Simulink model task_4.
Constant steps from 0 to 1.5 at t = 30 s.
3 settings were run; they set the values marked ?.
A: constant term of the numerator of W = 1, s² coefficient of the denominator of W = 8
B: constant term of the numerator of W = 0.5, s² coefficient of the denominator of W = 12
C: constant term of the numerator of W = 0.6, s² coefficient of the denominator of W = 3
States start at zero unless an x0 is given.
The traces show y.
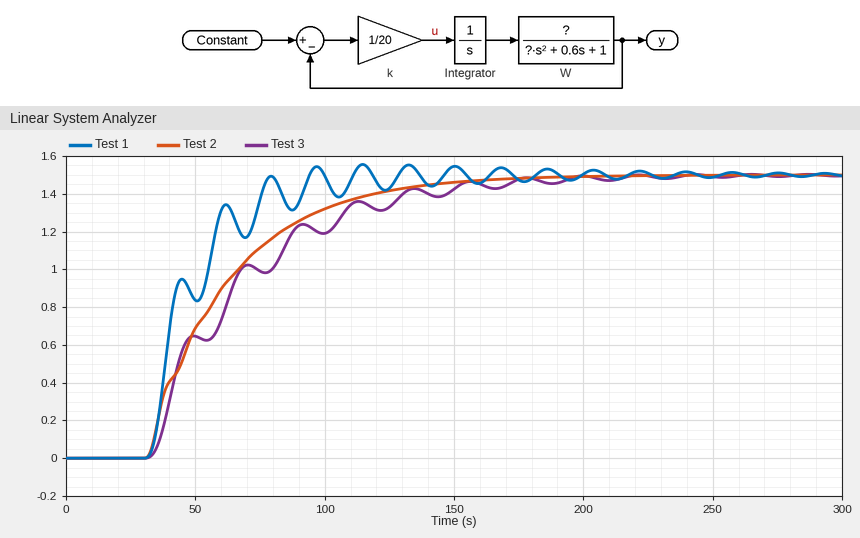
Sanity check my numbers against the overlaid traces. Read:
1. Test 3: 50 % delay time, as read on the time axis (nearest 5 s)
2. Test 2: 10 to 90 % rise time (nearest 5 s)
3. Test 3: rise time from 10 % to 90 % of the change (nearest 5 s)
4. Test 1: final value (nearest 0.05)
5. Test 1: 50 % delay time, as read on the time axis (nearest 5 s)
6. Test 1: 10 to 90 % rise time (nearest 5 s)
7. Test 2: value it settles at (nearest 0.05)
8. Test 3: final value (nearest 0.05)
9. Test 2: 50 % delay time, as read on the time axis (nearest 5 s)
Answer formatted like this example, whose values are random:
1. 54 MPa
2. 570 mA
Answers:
1. 60 s
2. 70 s
3. 75 s
4. 1.50
5. 40 s
6. 40 s
7. 1.50
8. 1.50
9. 55 s
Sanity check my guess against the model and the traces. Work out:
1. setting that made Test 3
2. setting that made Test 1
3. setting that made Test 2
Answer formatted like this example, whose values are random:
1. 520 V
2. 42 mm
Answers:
1. B
2. A
3. C
